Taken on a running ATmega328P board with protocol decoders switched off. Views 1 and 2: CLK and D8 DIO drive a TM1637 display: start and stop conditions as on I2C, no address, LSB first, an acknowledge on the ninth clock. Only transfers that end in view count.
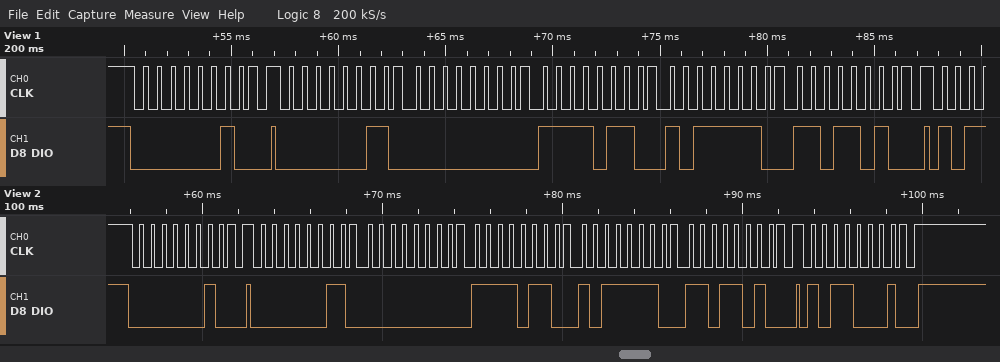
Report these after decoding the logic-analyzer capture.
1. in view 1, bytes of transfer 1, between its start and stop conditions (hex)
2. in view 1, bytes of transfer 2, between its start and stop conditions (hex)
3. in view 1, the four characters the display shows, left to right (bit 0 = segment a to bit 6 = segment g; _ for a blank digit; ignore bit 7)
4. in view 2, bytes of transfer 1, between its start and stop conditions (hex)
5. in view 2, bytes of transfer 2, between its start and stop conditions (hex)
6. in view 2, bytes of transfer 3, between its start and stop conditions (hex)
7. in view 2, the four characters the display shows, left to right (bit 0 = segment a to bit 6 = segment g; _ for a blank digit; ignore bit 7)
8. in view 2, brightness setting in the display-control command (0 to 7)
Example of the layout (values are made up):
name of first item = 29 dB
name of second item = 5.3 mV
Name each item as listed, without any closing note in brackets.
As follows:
in view 1, bytes of transfer 1, between its start and stop conditions = 40
in view 1, bytes of transfer 2, between its start and stop conditions = C0 00 6F 7D 5B
in view 1, the four characters the display shows, left to right = _962
in view 2, bytes of transfer 1, between its start and stop conditions = 40
in view 2, bytes of transfer 2, between its start and stop conditions = C0 00 6F 7D 5B
in view 2, bytes of transfer 3, between its start and stop conditions = 8D
in view 2, the four characters the display shows, left to right = _962
in view 2, brightness setting in the display-control command = 5
